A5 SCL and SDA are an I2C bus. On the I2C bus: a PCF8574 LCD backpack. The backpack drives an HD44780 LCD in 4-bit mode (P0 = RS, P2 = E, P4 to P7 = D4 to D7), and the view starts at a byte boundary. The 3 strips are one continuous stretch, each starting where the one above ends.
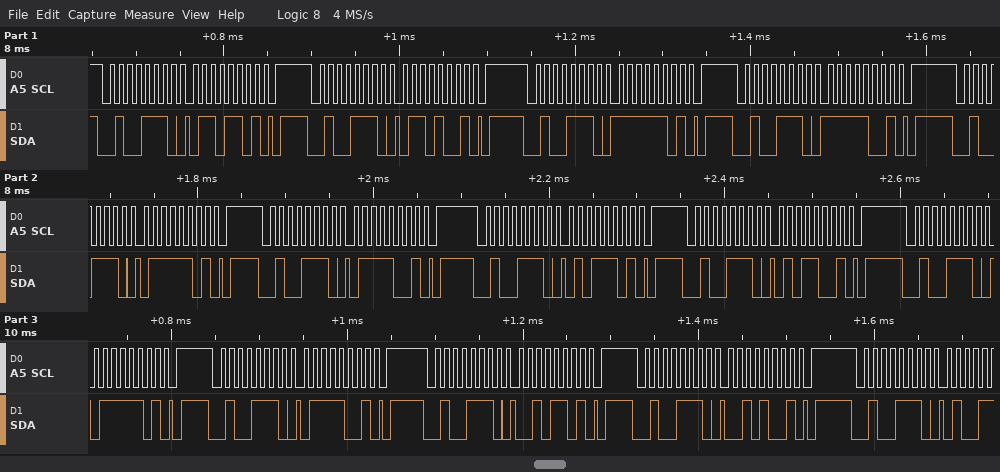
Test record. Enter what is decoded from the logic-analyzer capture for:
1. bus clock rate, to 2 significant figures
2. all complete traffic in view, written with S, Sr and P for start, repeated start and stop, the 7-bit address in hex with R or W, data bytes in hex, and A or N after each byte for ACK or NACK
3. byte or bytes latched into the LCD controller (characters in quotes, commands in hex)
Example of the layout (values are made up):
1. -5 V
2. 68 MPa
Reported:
1. 100 kHz
2. S 27W A 6D A P S 27W A 69 A P S 27W A FD A P S 27W A F9 A P S 27W A 7D A P S 27W A 79 A P S 27W A 5D A P S 27W A 59 A P S 27W A 7D A P S 27W A 79 A P S 27W A 2D A P S 27W A 29 A P S 27W A
3. 'o' 'u' 'r'
